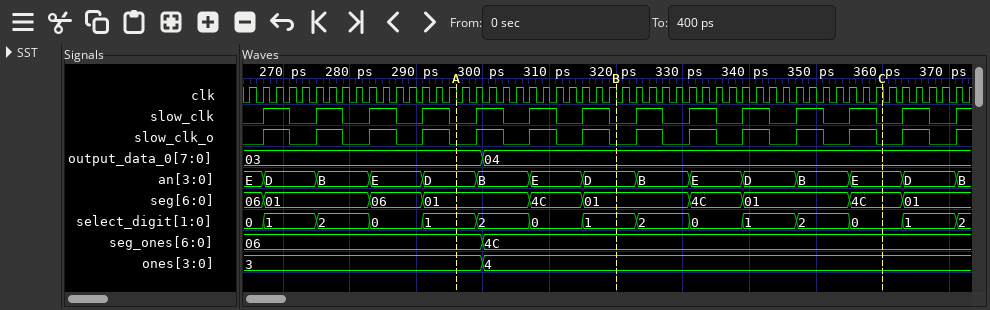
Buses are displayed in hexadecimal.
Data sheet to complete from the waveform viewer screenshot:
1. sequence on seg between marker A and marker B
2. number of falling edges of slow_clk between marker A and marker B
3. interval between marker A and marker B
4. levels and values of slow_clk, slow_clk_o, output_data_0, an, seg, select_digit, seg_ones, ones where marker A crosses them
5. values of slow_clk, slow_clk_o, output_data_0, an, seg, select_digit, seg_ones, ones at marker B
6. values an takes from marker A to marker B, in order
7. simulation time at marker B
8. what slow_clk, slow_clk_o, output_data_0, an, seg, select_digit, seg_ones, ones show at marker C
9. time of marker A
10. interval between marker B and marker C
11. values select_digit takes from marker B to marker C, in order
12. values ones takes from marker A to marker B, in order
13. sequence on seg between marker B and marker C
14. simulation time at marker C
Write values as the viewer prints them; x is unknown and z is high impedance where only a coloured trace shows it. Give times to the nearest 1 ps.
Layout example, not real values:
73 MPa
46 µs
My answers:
01, 4C, 01
3
24 ps
slow_clk=0, slow_clk_o=0, output_data_0=03, an=D, seg=01, select_digit=1, seg_ones=06, ones=3
slow_clk=0, slow_clk_o=0, output_data_0=04, an=D, seg=01, select_digit=1, seg_ones=4C, ones=4
D, B, E, D
320 ps
slow_clk=0, slow_clk_o=0, output_data_0=04, an=E, seg=4C, select_digit=0, seg_ones=4C, ones=4
296 ps
40 ps
1, 2, 0, 1, 2, 0
3, 4
01, 4C, 01, 4C
360 ps
